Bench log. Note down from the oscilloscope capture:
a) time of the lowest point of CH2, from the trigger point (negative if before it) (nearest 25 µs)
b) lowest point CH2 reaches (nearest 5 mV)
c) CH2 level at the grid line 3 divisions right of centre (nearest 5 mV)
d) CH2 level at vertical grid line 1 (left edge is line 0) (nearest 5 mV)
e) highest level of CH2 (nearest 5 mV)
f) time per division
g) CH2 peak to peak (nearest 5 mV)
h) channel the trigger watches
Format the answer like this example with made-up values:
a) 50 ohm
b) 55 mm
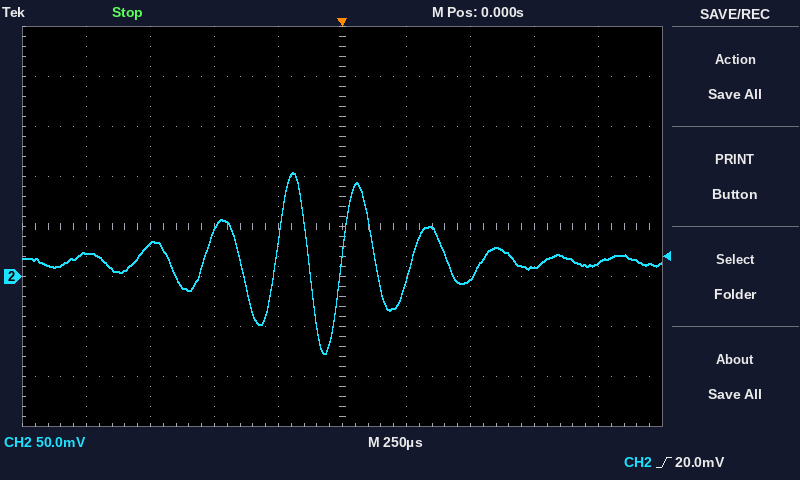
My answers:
a) -75 µs
b) -75 mV
c) 10 mV
d) 25 mV
e) 105 mV
f) 250 µs
g) 180 mV
h) CH2
